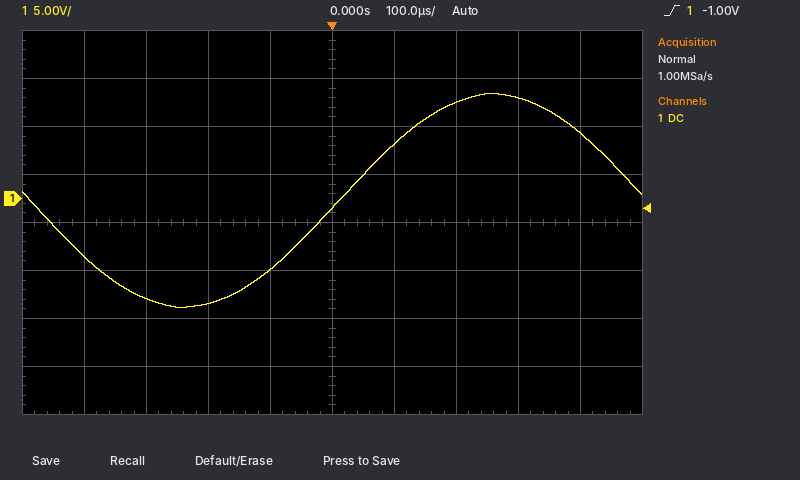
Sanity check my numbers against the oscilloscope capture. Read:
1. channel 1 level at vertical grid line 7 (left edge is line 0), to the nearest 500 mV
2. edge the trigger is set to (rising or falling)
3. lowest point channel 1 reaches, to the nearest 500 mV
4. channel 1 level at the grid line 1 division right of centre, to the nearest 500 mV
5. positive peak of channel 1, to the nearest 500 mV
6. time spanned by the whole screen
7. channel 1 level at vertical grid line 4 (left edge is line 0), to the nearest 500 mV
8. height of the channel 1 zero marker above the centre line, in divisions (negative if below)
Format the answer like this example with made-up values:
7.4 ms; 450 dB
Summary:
10.0 V; rising; -11.5 V; 5.5 V; 11.0 V; 1 ms; -7.5 V; +0.5 div
